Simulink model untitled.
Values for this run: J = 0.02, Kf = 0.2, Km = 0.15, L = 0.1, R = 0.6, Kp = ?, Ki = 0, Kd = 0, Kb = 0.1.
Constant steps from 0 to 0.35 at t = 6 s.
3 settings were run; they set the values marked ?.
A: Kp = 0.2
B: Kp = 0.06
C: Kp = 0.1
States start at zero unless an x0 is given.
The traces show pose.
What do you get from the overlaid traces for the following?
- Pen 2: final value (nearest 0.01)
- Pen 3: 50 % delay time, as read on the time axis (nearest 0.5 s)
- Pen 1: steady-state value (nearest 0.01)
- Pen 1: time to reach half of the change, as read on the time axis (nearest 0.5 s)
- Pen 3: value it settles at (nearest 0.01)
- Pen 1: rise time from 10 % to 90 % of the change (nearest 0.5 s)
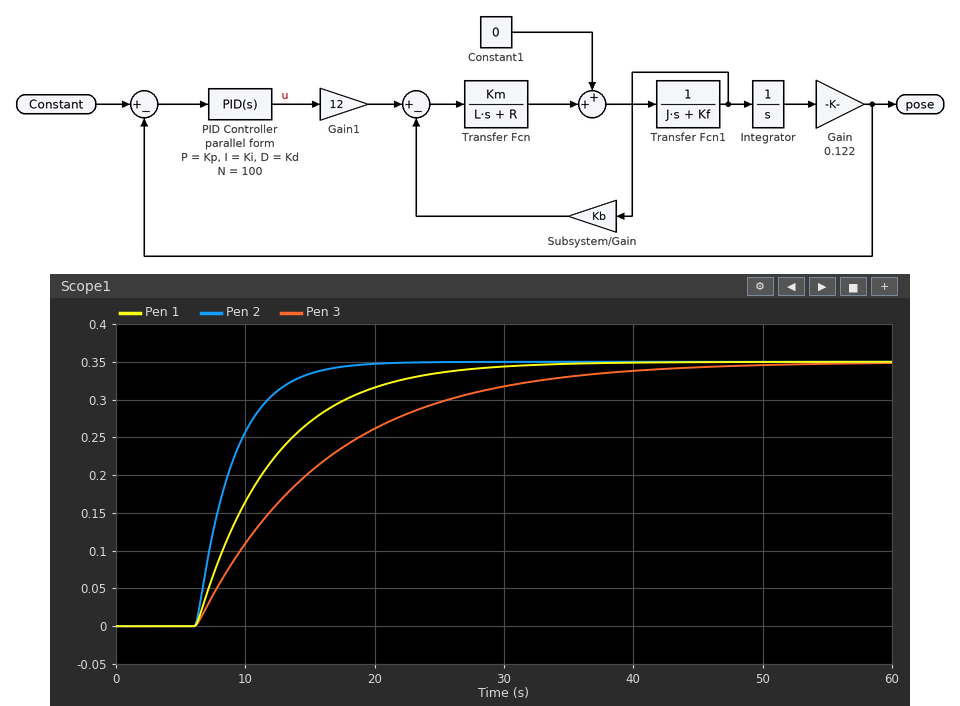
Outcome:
0.35
13.0 s
0.35
10.5 s
0.35
13.0 s
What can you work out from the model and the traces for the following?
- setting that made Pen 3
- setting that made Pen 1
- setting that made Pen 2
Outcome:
B
C
A
